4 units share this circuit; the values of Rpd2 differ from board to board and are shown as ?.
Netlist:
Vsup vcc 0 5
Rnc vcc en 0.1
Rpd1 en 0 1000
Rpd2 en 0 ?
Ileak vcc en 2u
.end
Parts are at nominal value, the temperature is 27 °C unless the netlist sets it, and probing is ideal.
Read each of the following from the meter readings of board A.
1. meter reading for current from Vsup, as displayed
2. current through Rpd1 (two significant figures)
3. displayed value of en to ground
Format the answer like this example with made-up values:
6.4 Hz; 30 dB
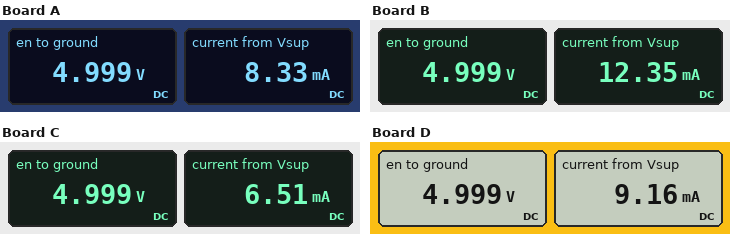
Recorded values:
8.33 mA; 5.0 mA; 4.999 V
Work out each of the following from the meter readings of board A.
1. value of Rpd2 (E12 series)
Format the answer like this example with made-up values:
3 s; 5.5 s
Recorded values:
1.5 kΩ
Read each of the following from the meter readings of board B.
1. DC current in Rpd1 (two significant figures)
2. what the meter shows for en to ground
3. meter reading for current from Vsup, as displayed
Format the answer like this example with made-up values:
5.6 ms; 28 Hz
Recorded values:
5.0 mA; 4.999 V; 12.35 mA
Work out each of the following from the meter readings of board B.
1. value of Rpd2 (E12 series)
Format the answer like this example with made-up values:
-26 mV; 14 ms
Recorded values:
680 Ω
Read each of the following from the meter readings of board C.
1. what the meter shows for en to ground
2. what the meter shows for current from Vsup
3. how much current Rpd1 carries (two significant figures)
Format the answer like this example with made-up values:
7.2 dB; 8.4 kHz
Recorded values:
4.999 V; 6.51 mA; 5.0 mA
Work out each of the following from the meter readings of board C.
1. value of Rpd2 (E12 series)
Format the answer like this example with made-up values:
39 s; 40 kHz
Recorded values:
3.3 kΩ
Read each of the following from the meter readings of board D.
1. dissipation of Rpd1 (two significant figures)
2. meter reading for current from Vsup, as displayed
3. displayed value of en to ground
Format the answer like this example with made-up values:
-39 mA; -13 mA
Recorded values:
25 mW; 9.16 mA; 4.999 V
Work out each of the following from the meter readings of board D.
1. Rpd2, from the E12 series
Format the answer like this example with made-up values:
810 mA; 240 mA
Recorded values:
1.2 kΩ
